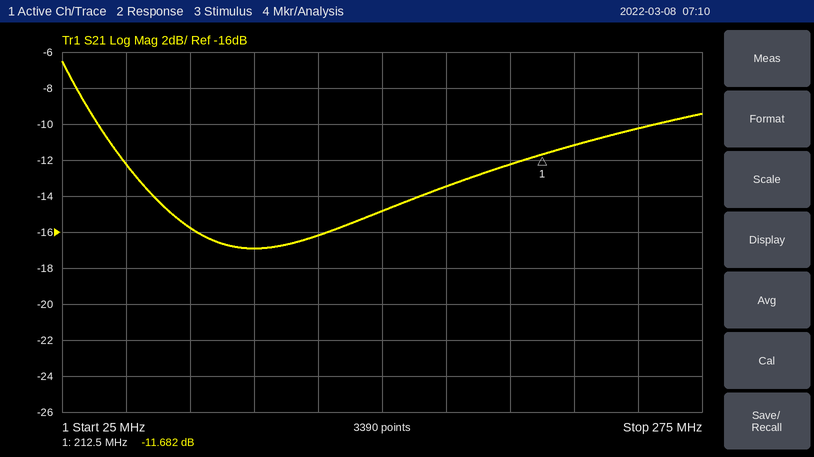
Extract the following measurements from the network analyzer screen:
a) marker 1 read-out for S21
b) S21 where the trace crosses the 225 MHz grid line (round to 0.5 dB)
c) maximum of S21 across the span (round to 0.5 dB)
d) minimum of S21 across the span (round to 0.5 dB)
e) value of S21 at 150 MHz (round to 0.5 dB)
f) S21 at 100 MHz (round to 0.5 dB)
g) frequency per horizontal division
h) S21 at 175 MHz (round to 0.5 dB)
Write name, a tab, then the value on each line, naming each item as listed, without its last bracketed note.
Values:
marker 1 read-out for S21	-11.682 dB
S21 where the trace crosses the 225 MHz grid line	-11.0 dB
maximum of S21 across the span	-6.5 dB
minimum of S21 across the span	-17.0 dB
value of S21 at 150 MHz	-15.0 dB
S21 at 100 MHz	-17.0 dB
frequency per horizontal division	25 MHz
S21 at 175 MHz	-13.5 dB
